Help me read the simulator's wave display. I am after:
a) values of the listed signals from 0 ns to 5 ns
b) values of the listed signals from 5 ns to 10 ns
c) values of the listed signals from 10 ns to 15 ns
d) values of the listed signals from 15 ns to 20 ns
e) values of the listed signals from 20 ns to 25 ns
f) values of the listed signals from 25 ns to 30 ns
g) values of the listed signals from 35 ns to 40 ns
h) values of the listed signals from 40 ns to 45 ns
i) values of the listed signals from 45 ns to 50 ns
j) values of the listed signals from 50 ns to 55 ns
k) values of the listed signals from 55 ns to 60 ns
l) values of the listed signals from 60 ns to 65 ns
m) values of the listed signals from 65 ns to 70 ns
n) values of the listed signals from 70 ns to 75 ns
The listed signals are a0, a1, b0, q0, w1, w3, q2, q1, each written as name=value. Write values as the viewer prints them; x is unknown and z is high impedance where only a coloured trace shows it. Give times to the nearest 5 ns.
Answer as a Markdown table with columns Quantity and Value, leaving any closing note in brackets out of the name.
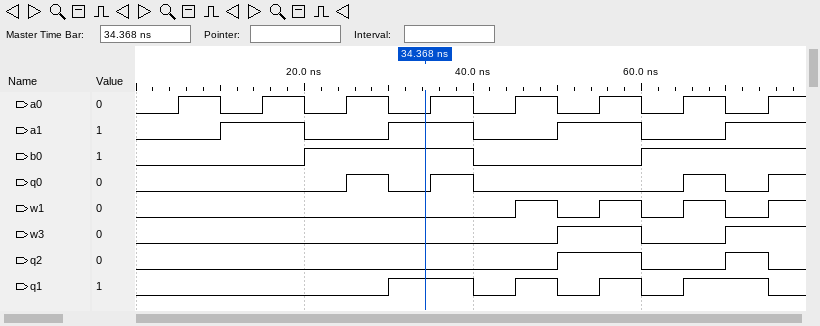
| Quantity | Value |
|---|---|
| values of the listed signals from 0 ns to 5 ns | a0=0, a1=0, b0=0, q0=0, w1=0, w3=0, q2=0, q1=0 |
| values of the listed signals from 5 ns to 10 ns | a0=1, a1=0, b0=0, q0=0, w1=0, w3=0, q2=0, q1=0 |
| values of the listed signals from 10 ns to 15 ns | a0=0, a1=1, b0=0, q0=0, w1=0, w3=0, q2=0, q1=0 |
| values of the listed signals from 15 ns to 20 ns | a0=1, a1=1, b0=0, q0=0, w1=0, w3=0, q2=0, q1=0 |
| values of the listed signals from 20 ns to 25 ns | a0=0, a1=0, b0=1, q0=0, w1=0, w3=0, q2=0, q1=0 |
| values of the listed signals from 25 ns to 30 ns | a0=1, a1=0, b0=1, q0=1, w1=0, w3=0, q2=0, q1=0 |
| values of the listed signals from 35 ns to 40 ns | a0=1, a1=1, b0=1, q0=1, w1=0, w3=0, q2=0, q1=1 |
| values of the listed signals from 40 ns to 45 ns | a0=0, a1=0, b0=0, q0=0, w1=0, w3=0, q2=0, q1=0 |
| values of the listed signals from 45 ns to 50 ns | a0=1, a1=0, b0=0, q0=0, w1=1, w3=0, q2=0, q1=1 |
| values of the listed signals from 50 ns to 55 ns | a0=0, a1=1, b0=0, q0=0, w1=0, w3=1, q2=1, q1=0 |
| values of the listed signals from 55 ns to 60 ns | a0=1, a1=1, b0=0, q0=0, w1=1, w3=1, q2=1, q1=1 |
| values of the listed signals from 60 ns to 65 ns | a0=0, a1=0, b0=1, q0=0, w1=0, w3=0, q2=0, q1=0 |
| values of the listed signals from 65 ns to 70 ns | a0=1, a1=0, b0=1, q0=1, w1=1, w3=0, q2=0, q1=1 |
| values of the listed signals from 70 ns to 75 ns | a0=0, a1=1, b0=1, q0=0, w1=0, w3=1, q2=1, q1=1 |
